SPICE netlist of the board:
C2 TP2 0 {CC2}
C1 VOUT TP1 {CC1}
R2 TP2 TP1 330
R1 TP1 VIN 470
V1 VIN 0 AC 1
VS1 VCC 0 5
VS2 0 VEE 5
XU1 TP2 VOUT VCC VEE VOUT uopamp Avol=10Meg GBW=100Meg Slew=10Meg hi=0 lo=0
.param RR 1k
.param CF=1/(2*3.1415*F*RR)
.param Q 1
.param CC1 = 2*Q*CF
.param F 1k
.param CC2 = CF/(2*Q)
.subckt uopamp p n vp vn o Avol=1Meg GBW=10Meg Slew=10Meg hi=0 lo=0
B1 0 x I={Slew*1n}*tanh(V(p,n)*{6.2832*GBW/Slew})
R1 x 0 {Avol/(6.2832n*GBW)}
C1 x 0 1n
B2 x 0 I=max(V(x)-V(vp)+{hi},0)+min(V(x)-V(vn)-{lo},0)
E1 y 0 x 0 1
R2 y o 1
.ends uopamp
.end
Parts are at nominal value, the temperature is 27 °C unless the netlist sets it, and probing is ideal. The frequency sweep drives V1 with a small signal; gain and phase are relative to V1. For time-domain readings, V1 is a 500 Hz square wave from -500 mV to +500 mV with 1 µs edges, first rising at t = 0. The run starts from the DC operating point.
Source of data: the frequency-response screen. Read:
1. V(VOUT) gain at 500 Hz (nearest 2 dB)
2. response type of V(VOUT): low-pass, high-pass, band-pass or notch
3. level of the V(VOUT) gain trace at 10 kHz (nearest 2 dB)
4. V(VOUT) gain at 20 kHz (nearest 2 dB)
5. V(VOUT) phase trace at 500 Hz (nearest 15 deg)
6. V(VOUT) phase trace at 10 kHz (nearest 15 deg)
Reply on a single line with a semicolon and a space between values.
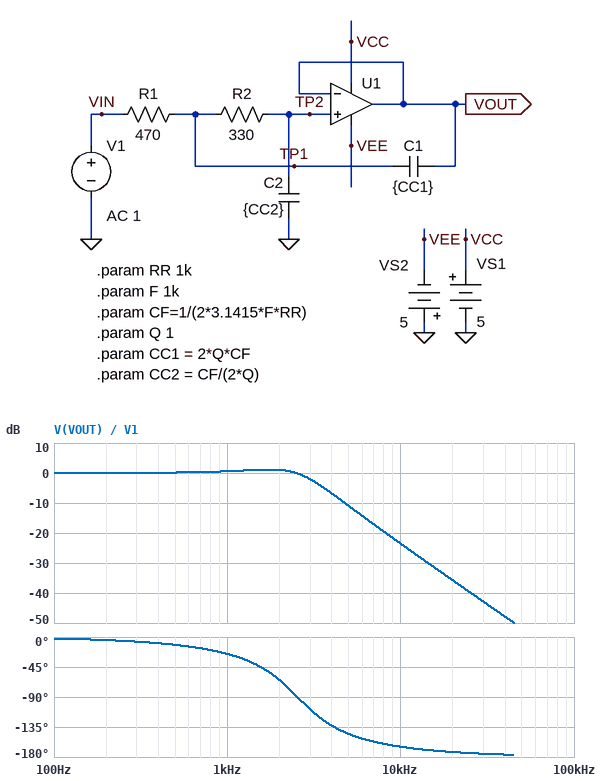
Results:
0 dB; low-pass; -24 dB; -36 dB; -15 deg; -165 deg
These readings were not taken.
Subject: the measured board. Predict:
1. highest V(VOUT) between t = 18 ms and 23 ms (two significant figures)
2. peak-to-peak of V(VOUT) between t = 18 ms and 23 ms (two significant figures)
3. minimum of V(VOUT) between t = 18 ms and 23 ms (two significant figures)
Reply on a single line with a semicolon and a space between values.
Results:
660 mV; 1.3 V; -660 mV
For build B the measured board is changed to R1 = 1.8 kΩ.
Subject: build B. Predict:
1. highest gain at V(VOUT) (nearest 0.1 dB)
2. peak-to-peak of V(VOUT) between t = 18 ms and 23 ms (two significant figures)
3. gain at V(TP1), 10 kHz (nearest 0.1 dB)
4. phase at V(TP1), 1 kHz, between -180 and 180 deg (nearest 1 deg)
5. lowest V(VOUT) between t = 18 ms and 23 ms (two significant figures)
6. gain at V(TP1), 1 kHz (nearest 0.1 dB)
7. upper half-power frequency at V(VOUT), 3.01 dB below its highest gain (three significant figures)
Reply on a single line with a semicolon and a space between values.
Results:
0 dB; 1.1 V; -29.8 dB; -60 deg; -550 mV; -1.0 dB; 1.33 kHz
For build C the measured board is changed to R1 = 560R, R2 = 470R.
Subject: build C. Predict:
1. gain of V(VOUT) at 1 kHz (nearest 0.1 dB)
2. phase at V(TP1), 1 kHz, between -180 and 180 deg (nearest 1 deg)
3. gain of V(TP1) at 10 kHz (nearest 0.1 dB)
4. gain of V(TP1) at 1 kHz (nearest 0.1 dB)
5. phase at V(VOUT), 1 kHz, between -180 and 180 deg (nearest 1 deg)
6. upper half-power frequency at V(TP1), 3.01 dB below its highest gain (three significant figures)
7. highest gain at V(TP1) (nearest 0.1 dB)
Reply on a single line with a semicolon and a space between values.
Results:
0.9 dB; -22 deg; -20.1 dB; 1.2 dB; -35 deg; 2.40 kHz; 1.7 dB
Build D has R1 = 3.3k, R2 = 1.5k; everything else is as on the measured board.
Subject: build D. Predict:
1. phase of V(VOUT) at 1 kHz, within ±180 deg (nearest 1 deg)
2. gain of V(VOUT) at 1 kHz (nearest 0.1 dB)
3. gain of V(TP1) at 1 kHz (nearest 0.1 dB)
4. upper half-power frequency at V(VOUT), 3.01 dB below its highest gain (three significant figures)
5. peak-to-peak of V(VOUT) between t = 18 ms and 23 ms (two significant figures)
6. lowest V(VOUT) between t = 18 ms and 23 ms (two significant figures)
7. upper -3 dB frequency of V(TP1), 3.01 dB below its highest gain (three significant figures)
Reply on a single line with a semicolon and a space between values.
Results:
-149 deg; -13.3 dB; -11.4 dB; 518 Hz; 1.1 V; -540 mV; 535 Hz
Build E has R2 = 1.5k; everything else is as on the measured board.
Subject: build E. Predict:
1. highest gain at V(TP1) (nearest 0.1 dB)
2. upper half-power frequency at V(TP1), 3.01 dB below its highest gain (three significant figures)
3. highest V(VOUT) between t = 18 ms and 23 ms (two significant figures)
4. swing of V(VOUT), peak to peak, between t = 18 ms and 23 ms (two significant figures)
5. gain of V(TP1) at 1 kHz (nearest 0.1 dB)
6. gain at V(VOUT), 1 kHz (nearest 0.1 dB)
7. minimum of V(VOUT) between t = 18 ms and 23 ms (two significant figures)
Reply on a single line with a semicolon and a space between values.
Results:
1.8 dB; 1.63 kHz; 600 mV; 1.2 V; 1.7 dB; -0.2 dB; -600 mV
